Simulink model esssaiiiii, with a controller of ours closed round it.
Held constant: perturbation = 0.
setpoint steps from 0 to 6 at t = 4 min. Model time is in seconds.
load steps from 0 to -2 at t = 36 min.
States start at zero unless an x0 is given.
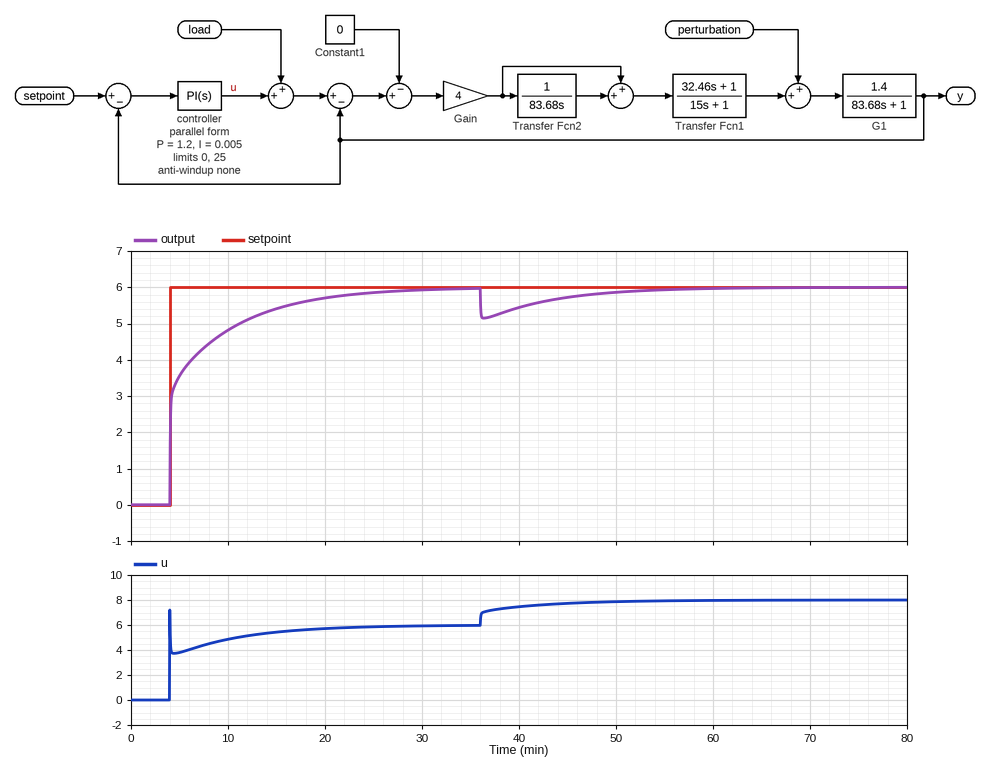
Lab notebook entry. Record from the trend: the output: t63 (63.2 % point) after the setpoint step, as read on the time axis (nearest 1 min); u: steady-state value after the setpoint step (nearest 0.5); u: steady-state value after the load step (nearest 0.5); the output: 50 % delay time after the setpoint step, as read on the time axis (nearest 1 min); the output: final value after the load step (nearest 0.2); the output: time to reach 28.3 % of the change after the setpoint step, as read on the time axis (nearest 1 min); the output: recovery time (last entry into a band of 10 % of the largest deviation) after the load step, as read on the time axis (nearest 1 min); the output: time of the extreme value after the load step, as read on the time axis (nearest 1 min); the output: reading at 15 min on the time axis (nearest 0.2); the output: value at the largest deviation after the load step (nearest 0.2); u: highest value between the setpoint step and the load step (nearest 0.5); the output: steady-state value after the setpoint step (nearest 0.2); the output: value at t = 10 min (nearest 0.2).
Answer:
6 min
6.0
8.0
4 min
6.0
4 min
54 min
36 min
5.4
5.2
7.0
6.0
4.8
